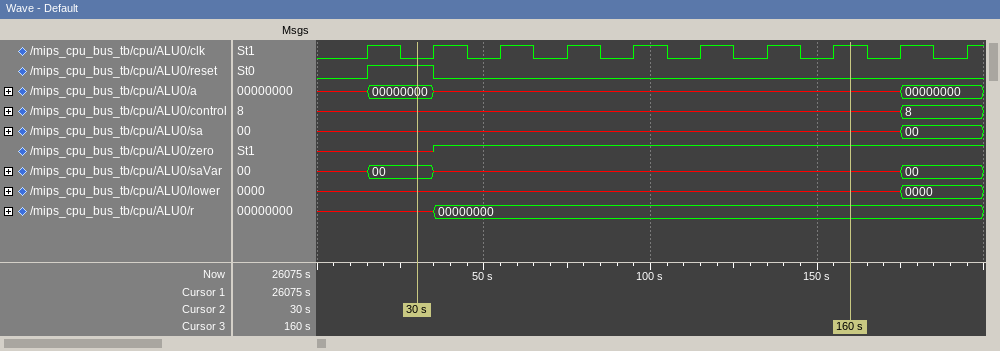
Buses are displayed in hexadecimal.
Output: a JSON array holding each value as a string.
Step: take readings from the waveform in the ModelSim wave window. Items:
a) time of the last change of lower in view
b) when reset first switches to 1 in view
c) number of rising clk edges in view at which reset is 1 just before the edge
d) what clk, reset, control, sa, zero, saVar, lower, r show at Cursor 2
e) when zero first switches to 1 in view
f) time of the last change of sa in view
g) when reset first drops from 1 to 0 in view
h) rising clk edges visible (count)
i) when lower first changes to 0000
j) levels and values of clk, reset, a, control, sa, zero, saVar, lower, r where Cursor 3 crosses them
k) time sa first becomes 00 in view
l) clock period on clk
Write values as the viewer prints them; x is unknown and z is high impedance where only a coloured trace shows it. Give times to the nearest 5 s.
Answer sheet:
["175 s", "15 s", "1", "clk=0, reset=1, control=x, sa=x, zero=x, saVar=00, lower=x, r=x", "35 s", "175 s", "35 s", "10", "175 s", "clk=1, reset=0, a=x, control=x, sa=x, zero=1, saVar=x, lower=x, r=00000000", "175 s", "20 s"]
